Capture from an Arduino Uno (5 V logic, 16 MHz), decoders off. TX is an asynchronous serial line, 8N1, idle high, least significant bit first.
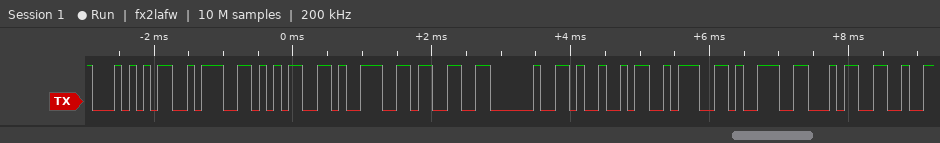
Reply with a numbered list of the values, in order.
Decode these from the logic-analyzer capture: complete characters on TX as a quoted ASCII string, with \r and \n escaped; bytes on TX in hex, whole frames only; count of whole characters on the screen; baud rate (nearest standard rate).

1. "T:593 I:94"
2. 54 3A 35 39 33 20 49 3A 39 34
3. 10
4. 9600 baud
